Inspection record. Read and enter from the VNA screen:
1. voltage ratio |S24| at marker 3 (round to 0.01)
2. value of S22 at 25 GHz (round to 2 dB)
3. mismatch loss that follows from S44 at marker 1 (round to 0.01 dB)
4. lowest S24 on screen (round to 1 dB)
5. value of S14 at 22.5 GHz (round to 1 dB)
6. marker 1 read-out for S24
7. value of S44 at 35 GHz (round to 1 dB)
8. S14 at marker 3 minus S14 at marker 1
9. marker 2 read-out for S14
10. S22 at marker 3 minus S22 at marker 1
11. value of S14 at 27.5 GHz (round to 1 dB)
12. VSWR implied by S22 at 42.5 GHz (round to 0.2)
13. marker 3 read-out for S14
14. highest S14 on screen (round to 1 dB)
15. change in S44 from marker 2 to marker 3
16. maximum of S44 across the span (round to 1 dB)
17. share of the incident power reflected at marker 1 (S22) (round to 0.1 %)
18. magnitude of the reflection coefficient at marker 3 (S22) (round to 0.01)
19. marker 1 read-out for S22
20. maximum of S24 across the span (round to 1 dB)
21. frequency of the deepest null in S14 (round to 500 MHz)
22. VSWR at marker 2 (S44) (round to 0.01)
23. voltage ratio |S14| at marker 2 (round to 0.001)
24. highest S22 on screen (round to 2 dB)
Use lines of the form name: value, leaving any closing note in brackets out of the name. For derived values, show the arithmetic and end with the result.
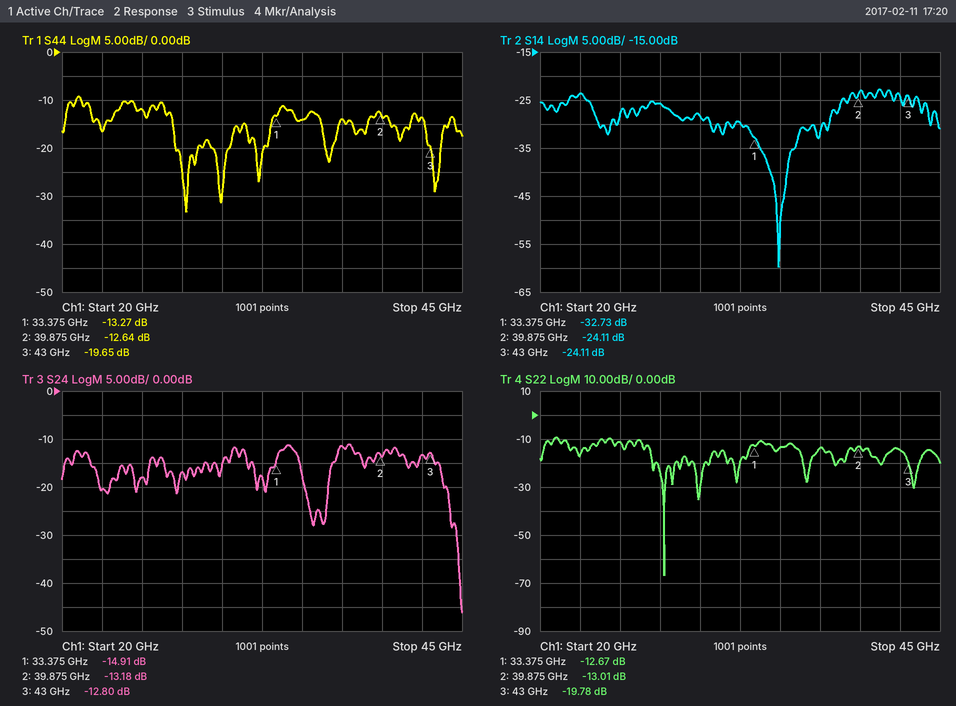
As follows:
voltage ratio |S24| at marker 3: 10^(-12.8/20) ≈ 0.23
value of S22 at 25 GHz: -12 dB
mismatch loss that follows from S44 at marker 1: −10 log10(1 − 10^(-13.27/10)) ≈ 0.21 dB
lowest S24 on screen: -46 dB
value of S14 at 22.5 GHz: -24 dB
marker 1 read-out for S24: -14.91 dB
value of S44 at 35 GHz: -14 dB
S14 at marker 3 minus S14 at marker 1: -24.11 − (-32.73) = 8.62 dB
marker 2 read-out for S14: -24.11 dB
S22 at marker 3 minus S22 at marker 1: -19.78 − (-12.67) = -7.11 dB
value of S14 at 27.5 GHz: -26 dB
VSWR implied by S22 at 42.5 GHz: |Γ| = 10^(-14/20) = 0.1995; VSWR = (1 + 0.1995)/(1 − 0.1995) ≈ 1.50, so 1.4 to the nearest 0.2
marker 3 read-out for S14: -24.11 dB
highest S14 on screen: -23 dB
change in S44 from marker 2 to marker 3: -19.65 − (-12.64) = -7.01 dB
maximum of S44 across the span: -9 dB
share of the incident power reflected at marker 1 (S22): 10^(-12.67/10) ≈ 5.4 %
magnitude of the reflection coefficient at marker 3 (S22): 10^(-19.78/20) ≈ 0.10
marker 1 read-out for S22: -12.67 dB
maximum of S24 across the span: -11 dB
frequency of the deepest null in S14: 35.0 GHz
VSWR at marker 2 (S44): (1 + 0.2333)/(1 − 0.2333) ≈ 1.61
voltage ratio |S14| at marker 2: 10^(-24.11/20) ≈ 0.062
highest S22 on screen: -10 dB
